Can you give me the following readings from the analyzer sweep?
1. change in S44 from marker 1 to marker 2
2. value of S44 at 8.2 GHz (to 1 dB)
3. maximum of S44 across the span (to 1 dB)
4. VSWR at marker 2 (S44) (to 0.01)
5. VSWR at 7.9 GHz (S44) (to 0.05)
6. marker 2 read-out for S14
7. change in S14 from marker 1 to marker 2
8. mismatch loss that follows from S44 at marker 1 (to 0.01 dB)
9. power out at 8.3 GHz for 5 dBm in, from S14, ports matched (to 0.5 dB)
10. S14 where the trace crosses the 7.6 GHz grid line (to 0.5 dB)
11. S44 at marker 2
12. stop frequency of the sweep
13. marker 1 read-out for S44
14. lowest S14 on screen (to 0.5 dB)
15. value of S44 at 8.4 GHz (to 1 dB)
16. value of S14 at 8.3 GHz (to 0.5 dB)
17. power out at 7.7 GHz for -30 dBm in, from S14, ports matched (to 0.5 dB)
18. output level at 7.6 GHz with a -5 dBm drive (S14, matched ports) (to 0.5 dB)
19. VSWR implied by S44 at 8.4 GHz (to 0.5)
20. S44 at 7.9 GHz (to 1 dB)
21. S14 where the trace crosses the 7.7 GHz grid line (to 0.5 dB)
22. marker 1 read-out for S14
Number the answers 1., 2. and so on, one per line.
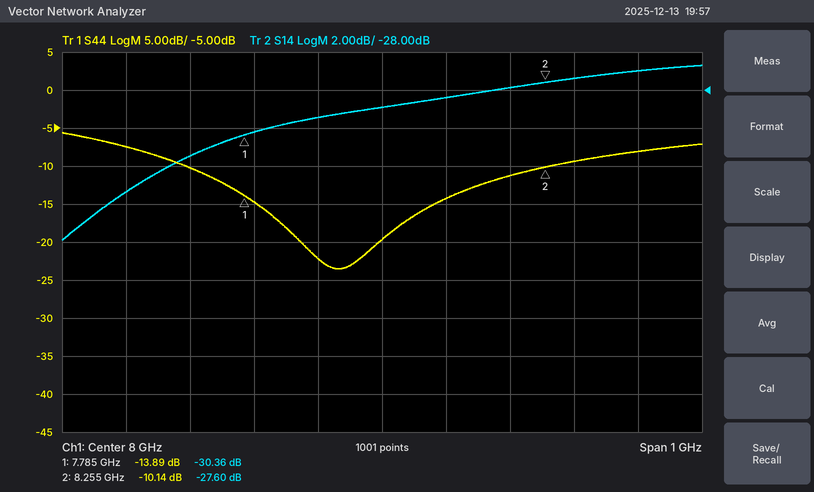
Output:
1. 3.75 dB
2. -11 dB
3. -6 dB
4. 1.90
5. 1.15
6. -27.60 dB
7. 2.76 dB
8. 0.18 dB
9. -22.5 dBm
10. -33.5 dB
11. -10.14 dB
12. 8.5 GHz
13. -13.89 dB
14. -36.0 dB
15. -8 dB
16. -27.5 dB
17. -61.5 dBm
18. -38.5 dBm
19. 2.5
20. -22 dB
21. -31.5 dB
22. -30.36 dB
